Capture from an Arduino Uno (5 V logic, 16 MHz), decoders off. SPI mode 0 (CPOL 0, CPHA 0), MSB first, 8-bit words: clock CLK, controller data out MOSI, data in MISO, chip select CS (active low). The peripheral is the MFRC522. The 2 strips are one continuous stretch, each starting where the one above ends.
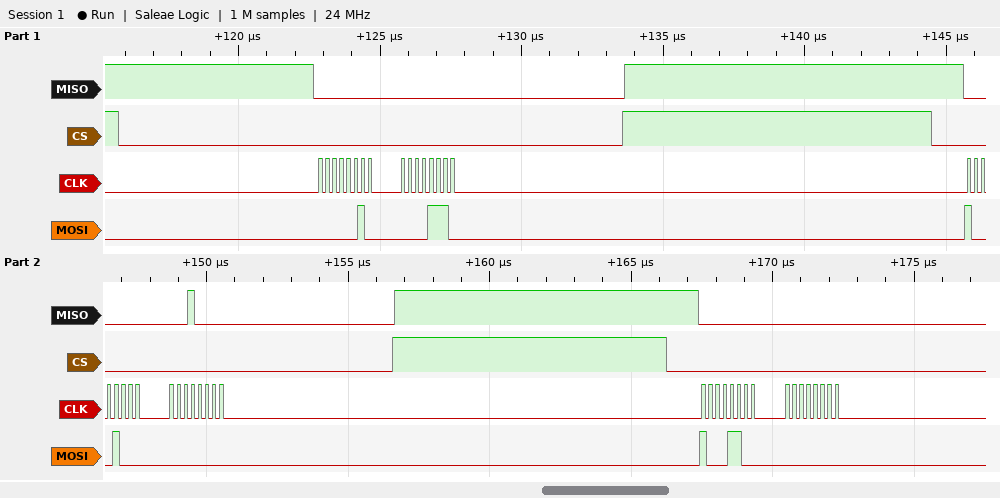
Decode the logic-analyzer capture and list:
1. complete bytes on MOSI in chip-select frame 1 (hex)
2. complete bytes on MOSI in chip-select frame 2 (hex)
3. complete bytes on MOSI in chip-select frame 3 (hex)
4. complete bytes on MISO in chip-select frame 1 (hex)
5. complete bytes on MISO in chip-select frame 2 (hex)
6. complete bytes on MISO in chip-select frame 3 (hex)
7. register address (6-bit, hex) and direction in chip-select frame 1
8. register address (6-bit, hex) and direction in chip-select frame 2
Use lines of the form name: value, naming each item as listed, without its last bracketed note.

complete bytes on MOSI in chip-select frame 1: 0x02 0x0E
complete bytes on MOSI in chip-select frame 2: 0x88 0x00
complete bytes on MOSI in chip-select frame 3: 0x8C 0x00
complete bytes on MISO in chip-select frame 1: 0x00 0x00
complete bytes on MISO in chip-select frame 2: 0x00 0x10
complete bytes on MISO in chip-select frame 3: 0x00 0x00
register address (6-bit, hex) and direction in chip-select frame 1: 0x01 write
register address (6-bit, hex) and direction in chip-select frame 2: 0x04 read
